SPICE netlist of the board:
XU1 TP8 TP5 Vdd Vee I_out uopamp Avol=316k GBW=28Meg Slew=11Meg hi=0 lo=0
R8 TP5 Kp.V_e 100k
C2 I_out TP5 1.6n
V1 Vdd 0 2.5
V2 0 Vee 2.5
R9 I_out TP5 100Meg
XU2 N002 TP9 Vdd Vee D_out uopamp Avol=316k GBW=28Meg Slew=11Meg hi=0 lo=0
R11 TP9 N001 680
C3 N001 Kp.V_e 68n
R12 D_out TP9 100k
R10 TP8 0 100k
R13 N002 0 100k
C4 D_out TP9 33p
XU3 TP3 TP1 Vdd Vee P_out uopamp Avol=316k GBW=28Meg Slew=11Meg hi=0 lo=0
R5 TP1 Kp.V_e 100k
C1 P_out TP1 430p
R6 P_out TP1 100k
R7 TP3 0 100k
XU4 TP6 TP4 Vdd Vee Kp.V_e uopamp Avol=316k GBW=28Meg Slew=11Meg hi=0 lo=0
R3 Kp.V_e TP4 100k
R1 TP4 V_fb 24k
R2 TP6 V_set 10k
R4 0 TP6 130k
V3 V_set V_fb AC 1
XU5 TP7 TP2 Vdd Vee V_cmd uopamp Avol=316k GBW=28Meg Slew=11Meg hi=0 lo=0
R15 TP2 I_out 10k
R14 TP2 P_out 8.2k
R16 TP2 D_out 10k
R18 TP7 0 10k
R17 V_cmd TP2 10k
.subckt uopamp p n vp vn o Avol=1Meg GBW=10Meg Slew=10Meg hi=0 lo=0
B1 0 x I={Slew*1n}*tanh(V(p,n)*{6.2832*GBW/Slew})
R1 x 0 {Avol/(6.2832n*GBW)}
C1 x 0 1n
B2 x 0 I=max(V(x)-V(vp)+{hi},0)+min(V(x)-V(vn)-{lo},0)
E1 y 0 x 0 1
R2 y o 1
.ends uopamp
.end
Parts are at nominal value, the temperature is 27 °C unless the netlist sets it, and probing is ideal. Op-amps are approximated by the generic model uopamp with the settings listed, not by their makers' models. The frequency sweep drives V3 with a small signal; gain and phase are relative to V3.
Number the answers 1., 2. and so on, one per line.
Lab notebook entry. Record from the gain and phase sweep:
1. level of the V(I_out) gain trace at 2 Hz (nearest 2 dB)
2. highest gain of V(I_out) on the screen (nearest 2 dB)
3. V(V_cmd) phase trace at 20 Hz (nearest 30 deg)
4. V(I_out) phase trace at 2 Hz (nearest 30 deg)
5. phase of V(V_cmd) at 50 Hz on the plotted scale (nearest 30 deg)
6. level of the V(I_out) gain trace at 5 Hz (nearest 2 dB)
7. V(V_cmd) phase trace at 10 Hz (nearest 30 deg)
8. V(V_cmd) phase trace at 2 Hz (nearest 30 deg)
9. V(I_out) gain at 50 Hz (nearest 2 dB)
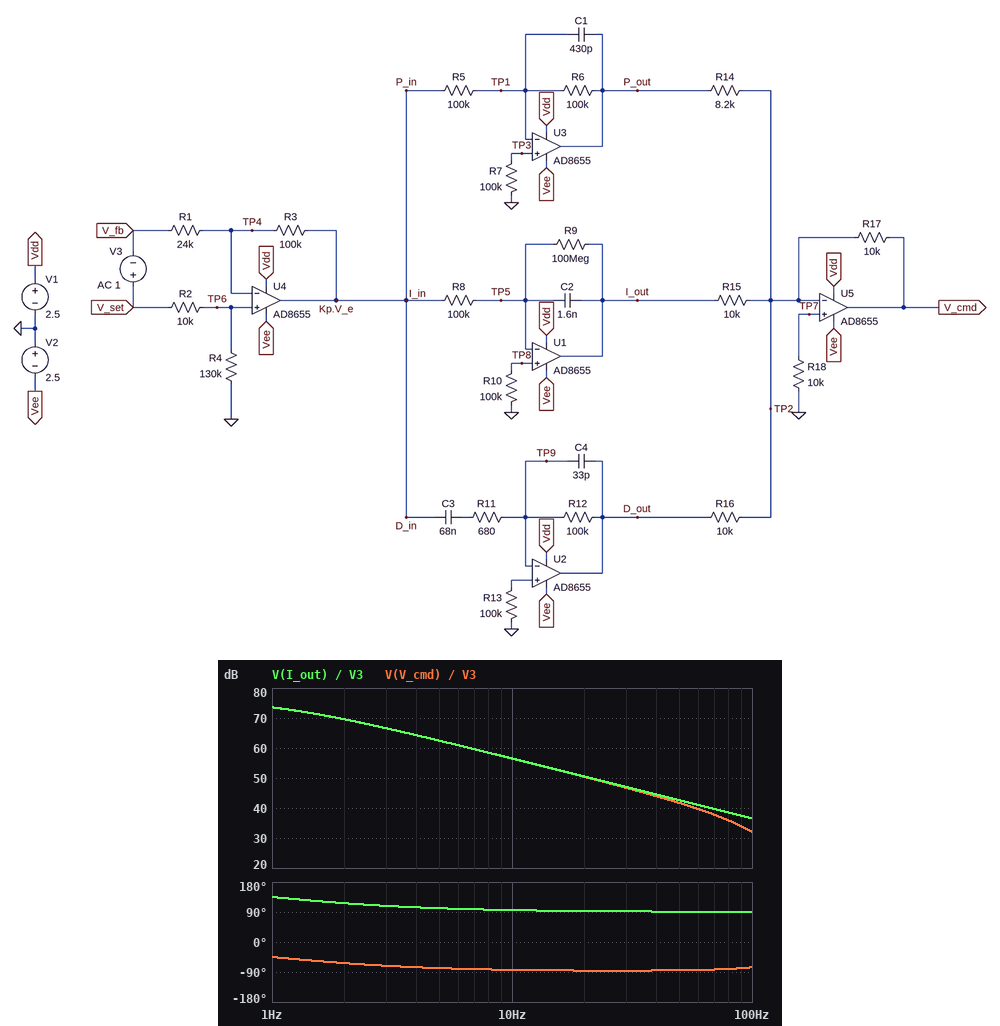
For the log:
1. 70 dB
2. 74 dB
3. -90 deg
4. 120 deg
5. -90 deg
6. 62 dB
7. -90 deg
8. -60 deg
9. 42 dB
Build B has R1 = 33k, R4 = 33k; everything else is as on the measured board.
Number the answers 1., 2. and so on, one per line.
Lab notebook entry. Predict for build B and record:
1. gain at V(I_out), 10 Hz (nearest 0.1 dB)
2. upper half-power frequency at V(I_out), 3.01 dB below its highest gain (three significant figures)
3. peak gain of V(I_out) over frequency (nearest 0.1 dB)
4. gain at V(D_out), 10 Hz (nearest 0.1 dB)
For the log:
1. 49.7 dB
2. 998 mHz
3. 69.8 dB
4. 2.4 dB
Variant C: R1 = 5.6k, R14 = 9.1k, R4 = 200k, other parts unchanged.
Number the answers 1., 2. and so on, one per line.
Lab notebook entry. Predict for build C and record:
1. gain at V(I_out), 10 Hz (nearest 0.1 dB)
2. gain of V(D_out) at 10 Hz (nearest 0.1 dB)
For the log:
1. 65.6 dB
2. 18.3 dB
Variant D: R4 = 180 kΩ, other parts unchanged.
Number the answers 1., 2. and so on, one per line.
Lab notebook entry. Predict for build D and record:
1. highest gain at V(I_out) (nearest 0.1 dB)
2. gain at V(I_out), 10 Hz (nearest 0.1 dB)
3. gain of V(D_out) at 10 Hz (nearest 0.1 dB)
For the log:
1. 78.3 dB
2. 58.2 dB
3. 10.9 dB
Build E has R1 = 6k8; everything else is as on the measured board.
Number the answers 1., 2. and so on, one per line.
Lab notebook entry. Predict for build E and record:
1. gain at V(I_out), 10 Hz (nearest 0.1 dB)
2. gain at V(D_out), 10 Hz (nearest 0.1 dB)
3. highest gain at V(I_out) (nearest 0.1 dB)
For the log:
1. 62.6 dB
2. 15.3 dB
3. 82.7 dB
